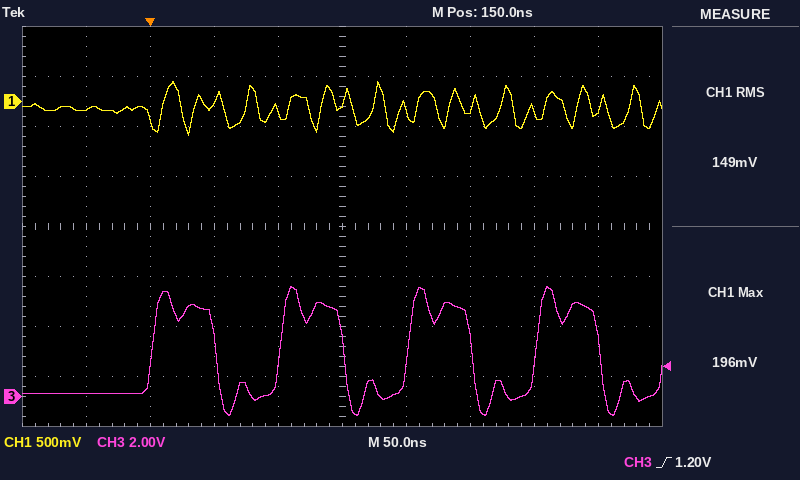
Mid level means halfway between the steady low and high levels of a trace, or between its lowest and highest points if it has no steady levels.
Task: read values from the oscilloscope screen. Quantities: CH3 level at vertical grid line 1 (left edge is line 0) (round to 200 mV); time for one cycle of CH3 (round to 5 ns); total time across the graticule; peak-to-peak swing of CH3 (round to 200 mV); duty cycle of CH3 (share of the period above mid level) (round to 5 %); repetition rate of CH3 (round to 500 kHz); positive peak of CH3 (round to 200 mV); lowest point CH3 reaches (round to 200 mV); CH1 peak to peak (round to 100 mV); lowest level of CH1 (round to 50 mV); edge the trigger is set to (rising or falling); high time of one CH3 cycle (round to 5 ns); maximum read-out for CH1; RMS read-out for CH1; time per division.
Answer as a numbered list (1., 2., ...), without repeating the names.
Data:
1. 200 mV
2. 100 ns
3. 500 ns
4. 5.2 V
5. 50 %
6. 10.0 MHz
7. 4.4 V
8. -800 mV
9. 500 mV
10. -350 mV
11. rising
12. 50 ns
13. 196 mV
14. 149 mV
15. 50 ns
